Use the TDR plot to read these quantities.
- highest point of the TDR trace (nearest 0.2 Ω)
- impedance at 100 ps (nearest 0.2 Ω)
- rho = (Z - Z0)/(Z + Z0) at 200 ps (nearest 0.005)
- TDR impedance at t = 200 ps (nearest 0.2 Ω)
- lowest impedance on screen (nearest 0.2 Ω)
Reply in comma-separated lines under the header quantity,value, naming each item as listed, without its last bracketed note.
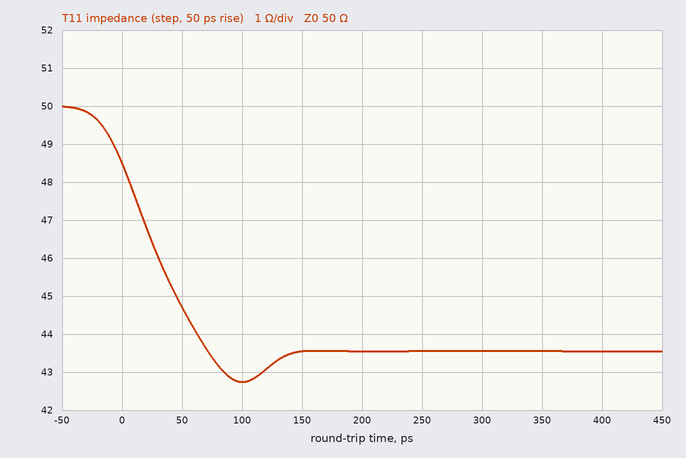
quantity,value
highest point of the TDR trace,50.0 Ω
impedance at 100 ps,42.8 Ω
rho = (Z - Z0)/(Z + Z0) at 200 ps,-0.070
TDR impedance at t = 200 ps,43.6 Ω
lowest impedance on screen,42.8 Ω
